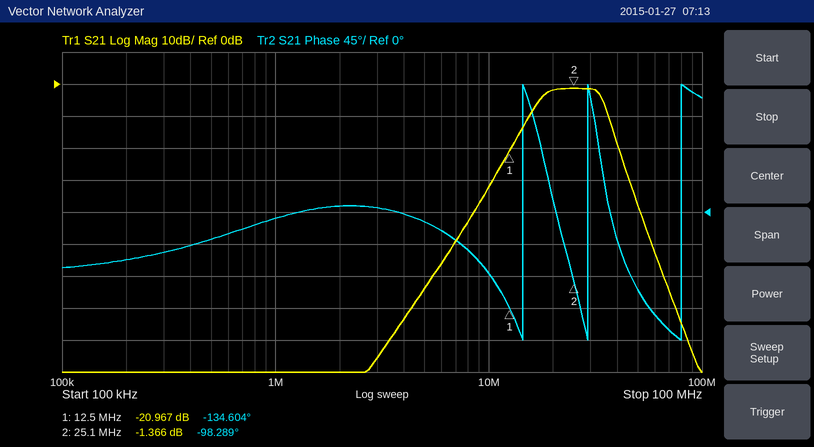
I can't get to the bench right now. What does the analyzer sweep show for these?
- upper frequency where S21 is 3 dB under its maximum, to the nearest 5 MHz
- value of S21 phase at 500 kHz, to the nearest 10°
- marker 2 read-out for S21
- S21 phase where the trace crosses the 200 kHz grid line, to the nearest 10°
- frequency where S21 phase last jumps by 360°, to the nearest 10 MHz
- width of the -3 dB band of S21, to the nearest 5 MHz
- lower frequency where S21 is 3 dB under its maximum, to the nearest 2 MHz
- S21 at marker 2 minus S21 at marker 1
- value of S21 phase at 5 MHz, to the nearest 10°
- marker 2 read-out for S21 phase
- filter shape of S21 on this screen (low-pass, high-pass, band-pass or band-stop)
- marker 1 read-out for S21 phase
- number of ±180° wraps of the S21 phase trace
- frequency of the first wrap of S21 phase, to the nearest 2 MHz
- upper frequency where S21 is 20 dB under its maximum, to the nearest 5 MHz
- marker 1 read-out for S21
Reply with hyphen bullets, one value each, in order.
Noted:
- 35 MHz
- -40°
- -1.366 dB
- -70°
- 80 MHz
- 15 MHz
- 18 MHz
- 19.601 dB
- -10°
- -98.289°
- band-pass
- -134.604°
- 3
- 14 MHz
- 40 MHz
- -20.967 dB
